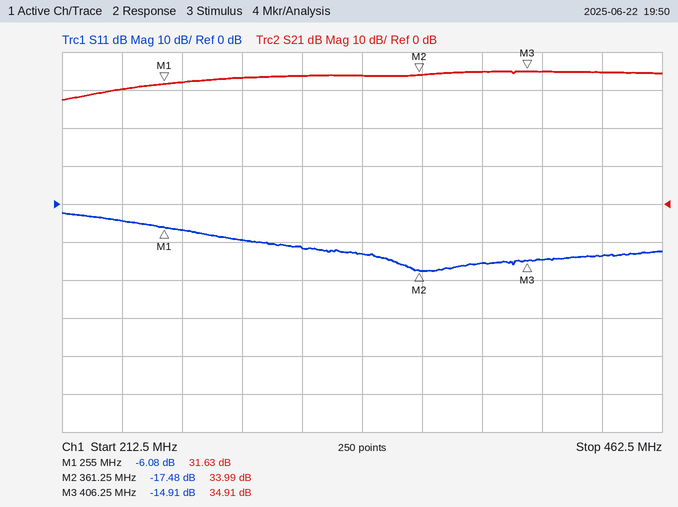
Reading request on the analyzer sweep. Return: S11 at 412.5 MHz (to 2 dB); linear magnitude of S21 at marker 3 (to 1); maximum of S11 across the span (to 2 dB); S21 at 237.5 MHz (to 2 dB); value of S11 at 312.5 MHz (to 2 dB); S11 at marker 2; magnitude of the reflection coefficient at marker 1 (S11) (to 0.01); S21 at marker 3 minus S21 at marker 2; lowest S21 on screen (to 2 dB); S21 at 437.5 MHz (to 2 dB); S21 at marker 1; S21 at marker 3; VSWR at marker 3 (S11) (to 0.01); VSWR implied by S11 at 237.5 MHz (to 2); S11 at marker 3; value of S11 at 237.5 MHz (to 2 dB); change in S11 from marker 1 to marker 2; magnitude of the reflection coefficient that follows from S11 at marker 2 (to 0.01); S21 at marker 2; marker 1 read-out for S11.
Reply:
-14 dB
56
-2 dB
30 dB
-12 dB
-17.48 dB
0.50
0.92 dB
28 dB
34 dB
31.63 dB
34.91 dB
1.44
4
-14.91 dB
-4 dB
-11.40 dB
0.13
33.99 dB
-6.08 dB
